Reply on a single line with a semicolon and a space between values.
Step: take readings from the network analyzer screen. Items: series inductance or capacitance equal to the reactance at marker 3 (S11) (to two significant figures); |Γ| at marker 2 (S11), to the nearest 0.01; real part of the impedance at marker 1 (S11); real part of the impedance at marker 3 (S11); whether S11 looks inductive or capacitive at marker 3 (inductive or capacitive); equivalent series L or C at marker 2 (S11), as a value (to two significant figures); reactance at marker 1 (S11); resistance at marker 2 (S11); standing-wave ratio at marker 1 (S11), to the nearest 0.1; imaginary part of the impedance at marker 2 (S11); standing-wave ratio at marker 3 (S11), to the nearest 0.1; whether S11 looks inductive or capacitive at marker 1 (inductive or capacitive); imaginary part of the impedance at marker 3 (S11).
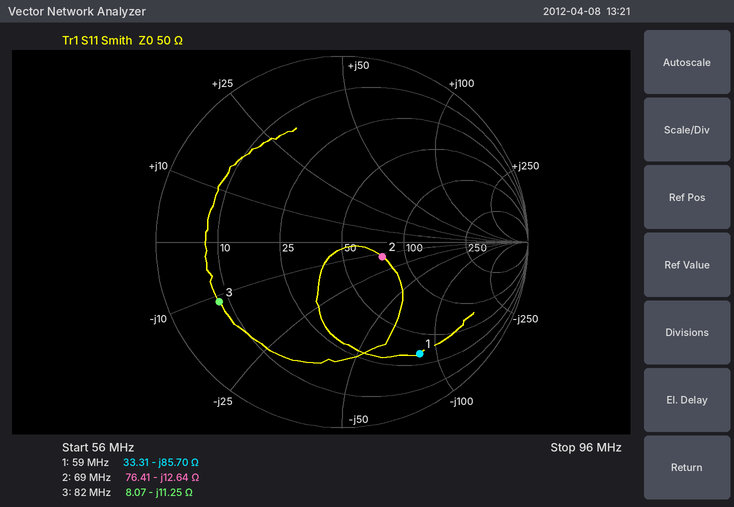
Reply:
170 pF; 0.23; 33.31 Ω; 8.07 Ω; capacitive; 180 pF; -85.70 Ω; 76.41 Ω; 6.4; -12.64 Ω; 6.5; capacitive; -11.25 Ω
